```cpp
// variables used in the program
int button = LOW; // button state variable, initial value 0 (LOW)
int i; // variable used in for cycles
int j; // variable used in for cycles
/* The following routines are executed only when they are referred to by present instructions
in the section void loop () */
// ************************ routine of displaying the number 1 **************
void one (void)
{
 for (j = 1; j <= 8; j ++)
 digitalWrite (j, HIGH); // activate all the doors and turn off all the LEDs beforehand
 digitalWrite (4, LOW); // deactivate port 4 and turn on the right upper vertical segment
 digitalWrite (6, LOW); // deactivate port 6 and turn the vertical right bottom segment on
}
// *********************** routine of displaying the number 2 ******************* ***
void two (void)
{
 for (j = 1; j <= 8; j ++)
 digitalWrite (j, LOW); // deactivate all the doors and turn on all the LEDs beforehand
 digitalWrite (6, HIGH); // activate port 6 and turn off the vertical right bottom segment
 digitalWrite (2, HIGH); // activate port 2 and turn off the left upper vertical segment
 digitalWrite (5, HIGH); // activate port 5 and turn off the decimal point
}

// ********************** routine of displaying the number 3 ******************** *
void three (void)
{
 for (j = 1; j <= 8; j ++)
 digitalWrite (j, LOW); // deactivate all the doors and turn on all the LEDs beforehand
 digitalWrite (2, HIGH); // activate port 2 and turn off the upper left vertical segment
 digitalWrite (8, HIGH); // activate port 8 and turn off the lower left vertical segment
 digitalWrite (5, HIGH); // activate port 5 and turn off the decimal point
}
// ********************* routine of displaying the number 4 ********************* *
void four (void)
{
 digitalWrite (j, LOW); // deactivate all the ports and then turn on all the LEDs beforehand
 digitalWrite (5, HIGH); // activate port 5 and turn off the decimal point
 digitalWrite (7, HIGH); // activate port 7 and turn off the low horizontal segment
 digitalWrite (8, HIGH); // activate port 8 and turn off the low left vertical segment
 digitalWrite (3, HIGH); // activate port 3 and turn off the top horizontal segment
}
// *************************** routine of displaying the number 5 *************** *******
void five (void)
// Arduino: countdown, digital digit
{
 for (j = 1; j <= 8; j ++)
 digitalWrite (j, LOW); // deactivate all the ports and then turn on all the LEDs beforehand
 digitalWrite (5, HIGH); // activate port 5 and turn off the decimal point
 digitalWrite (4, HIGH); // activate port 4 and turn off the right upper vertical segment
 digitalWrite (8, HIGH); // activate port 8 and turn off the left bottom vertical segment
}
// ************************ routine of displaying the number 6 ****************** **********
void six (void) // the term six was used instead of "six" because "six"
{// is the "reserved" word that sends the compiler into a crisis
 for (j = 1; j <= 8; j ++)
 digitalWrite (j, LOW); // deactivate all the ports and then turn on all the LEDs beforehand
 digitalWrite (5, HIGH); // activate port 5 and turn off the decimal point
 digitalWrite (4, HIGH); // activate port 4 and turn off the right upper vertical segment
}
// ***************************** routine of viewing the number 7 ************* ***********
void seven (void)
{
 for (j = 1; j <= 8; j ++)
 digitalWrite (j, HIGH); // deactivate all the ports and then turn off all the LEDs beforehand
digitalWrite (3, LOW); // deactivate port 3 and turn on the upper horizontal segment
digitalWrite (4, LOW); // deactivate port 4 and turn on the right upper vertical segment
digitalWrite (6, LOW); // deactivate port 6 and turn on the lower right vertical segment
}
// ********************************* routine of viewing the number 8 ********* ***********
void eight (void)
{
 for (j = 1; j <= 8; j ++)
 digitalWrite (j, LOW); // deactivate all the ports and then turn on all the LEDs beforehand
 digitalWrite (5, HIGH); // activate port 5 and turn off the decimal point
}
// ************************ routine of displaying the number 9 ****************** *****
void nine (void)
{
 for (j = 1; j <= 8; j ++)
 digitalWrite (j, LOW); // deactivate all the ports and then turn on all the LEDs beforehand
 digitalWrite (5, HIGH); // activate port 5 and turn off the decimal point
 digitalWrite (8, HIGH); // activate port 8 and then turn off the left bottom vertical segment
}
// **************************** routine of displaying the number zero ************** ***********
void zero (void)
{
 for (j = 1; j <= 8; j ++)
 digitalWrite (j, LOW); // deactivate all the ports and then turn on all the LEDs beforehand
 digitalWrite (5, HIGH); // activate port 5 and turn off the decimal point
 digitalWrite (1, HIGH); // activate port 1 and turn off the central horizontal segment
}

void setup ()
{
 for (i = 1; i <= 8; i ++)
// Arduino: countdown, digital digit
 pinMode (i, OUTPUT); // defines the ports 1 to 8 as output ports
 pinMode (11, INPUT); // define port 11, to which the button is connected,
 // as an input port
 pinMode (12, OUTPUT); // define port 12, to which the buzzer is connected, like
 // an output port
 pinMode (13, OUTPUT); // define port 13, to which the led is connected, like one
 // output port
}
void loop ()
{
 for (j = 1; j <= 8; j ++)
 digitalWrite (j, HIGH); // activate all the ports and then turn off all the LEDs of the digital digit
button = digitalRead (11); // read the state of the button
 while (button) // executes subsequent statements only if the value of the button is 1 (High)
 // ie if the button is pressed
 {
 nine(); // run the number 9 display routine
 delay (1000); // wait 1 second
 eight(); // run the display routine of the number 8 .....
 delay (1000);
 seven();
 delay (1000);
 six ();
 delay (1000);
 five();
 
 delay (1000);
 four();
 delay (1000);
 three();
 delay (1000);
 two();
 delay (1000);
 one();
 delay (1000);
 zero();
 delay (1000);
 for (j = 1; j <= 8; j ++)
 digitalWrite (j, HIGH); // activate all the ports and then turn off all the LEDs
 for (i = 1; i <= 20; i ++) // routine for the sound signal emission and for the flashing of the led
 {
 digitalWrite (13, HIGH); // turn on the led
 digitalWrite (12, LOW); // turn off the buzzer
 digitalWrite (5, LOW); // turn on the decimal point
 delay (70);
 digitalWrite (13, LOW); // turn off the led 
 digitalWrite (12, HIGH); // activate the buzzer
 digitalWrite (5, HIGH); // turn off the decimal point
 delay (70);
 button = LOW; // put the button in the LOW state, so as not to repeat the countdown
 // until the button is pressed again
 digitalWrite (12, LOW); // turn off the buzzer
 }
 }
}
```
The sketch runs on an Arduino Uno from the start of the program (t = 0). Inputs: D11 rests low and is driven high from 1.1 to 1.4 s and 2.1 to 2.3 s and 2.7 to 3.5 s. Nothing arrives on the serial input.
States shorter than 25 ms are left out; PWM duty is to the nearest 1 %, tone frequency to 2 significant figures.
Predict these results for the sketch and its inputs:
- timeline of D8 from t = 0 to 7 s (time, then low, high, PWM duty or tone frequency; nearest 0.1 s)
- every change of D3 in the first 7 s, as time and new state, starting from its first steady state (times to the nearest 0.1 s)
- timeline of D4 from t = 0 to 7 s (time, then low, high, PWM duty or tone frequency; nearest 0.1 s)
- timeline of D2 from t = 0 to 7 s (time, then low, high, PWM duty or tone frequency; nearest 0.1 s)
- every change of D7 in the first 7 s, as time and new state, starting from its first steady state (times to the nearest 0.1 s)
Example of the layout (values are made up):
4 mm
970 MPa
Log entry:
0 s high; 2.1 s low; 3.1 s high; 4.1 s low; 5.1 s high
0 s high; 1.1 s low; 6.1 s high
0 s high; 1.1 s low; 4.1 s high
0 s high; 1.1 s low; 3.1 s high; 4.1 s low
0 s high; 1.1 s low; 3.1 s high; 4.1 s low; 6.1 s high
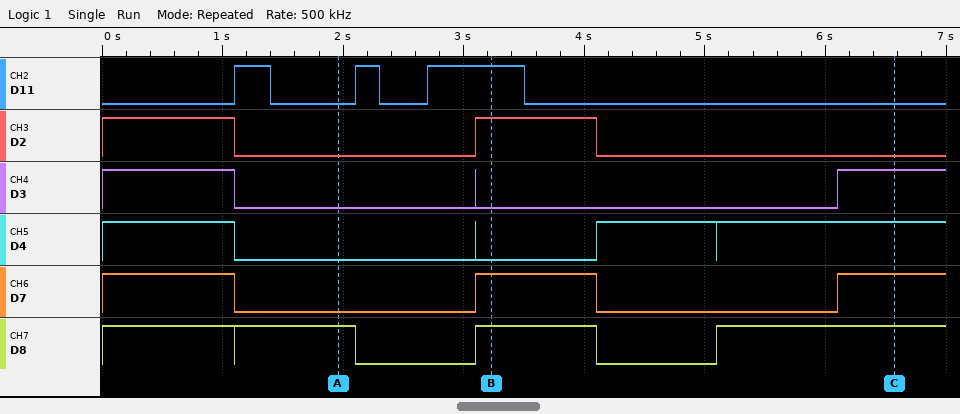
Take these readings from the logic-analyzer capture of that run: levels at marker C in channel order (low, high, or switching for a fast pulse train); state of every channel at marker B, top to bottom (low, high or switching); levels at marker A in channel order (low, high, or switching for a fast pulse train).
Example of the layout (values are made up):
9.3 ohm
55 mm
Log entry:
D11 low, D2 low, D3 high, D4 high, D7 high, D8 high
D11 high, D2 high, D3 low, D4 low, D7 high, D8 high
D11 low, D2 low, D3 low, D4 low, D7 low, D8 high
